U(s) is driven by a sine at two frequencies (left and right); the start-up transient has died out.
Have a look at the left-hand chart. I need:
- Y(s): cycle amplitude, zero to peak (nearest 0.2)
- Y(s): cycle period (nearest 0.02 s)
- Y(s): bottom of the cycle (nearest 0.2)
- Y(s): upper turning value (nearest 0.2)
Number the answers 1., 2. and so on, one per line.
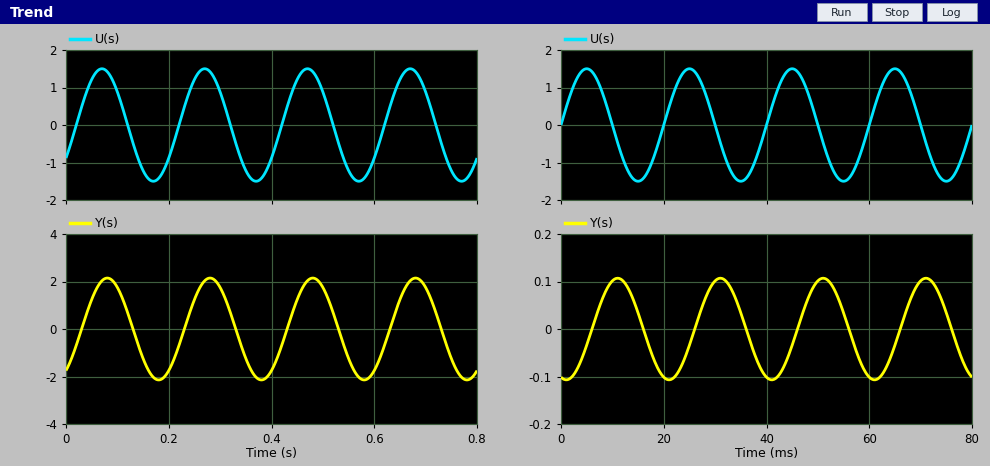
1. 2.2
2. 0.20 s
3. -2.2
4. 2.2
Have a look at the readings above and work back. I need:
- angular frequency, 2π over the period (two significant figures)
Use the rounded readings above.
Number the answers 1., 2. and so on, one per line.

1. 31 rad/s
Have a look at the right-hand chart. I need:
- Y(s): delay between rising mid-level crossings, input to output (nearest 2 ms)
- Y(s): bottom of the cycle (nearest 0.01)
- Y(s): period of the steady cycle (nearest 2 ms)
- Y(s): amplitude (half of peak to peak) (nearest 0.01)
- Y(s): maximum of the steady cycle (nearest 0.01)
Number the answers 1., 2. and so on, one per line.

1. 6 ms
2. -0.11
3. 20 ms
4. 0.11
5. 0.11
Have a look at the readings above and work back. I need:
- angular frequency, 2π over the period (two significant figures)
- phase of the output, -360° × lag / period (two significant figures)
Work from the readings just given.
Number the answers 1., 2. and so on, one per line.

1. 0.31 rad/ms
2. -110°
